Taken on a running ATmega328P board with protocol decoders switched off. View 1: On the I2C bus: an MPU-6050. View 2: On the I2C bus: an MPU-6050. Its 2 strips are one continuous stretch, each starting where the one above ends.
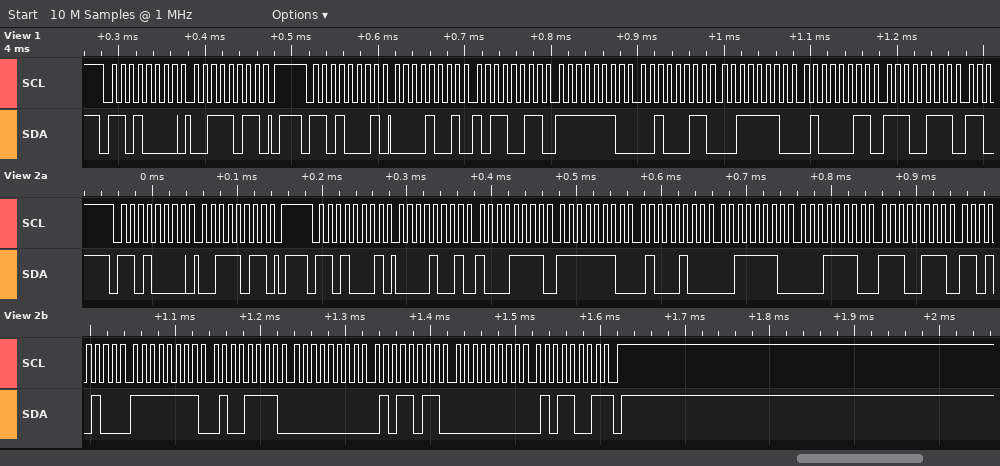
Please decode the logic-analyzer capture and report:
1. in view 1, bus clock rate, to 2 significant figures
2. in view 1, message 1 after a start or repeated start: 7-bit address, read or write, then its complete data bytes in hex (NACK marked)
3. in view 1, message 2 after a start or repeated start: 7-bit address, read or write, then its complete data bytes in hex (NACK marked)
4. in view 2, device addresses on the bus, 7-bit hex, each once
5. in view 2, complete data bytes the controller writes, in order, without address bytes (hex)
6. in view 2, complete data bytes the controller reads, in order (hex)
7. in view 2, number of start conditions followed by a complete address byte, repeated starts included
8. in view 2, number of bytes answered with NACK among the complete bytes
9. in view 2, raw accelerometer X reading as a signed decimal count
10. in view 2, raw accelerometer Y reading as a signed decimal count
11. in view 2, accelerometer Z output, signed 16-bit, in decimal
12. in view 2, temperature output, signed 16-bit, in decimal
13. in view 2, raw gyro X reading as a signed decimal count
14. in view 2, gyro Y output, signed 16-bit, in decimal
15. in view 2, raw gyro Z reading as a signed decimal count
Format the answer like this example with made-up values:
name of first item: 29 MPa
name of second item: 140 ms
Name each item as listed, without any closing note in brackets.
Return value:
in view 1, bus clock rate, to 2 significant figures: 100 kHz
in view 1, message 1 after a start or repeated start: 7-bit address, read or write, then its complete data bytes in hex: 0x68 write: 3B
in view 1, message 2 after a start or repeated start: 7-bit address, read or write, then its complete data bytes in hex: 0x68 read: 09 B3 FE 23 3E 43 E7
in view 2, device addresses on the bus, 7-bit hex, each once: 0x68
in view 2, complete data bytes the controller writes, in order, without address bytes: 3B
in view 2, complete data bytes the controller reads, in order: 09 8F FE 44 3E 1E E7 D4 FF 4F 00 5B 00 59
in view 2, number of start conditions followed by a complete address byte, repeated starts included: 2
in view 2, number of bytes answered with NACK among the complete bytes: 1
in view 2, raw accelerometer X reading as a signed decimal count: 2447
in view 2, raw accelerometer Y reading as a signed decimal count: -444
in view 2, accelerometer Z output, signed 16-bit, in decimal: 15902
in view 2, temperature output, signed 16-bit, in decimal: -6188
in view 2, raw gyro X reading as a signed decimal count: -177
in view 2, gyro Y output, signed 16-bit, in decimal: 91
in view 2, raw gyro Z reading as a signed decimal count: 89
